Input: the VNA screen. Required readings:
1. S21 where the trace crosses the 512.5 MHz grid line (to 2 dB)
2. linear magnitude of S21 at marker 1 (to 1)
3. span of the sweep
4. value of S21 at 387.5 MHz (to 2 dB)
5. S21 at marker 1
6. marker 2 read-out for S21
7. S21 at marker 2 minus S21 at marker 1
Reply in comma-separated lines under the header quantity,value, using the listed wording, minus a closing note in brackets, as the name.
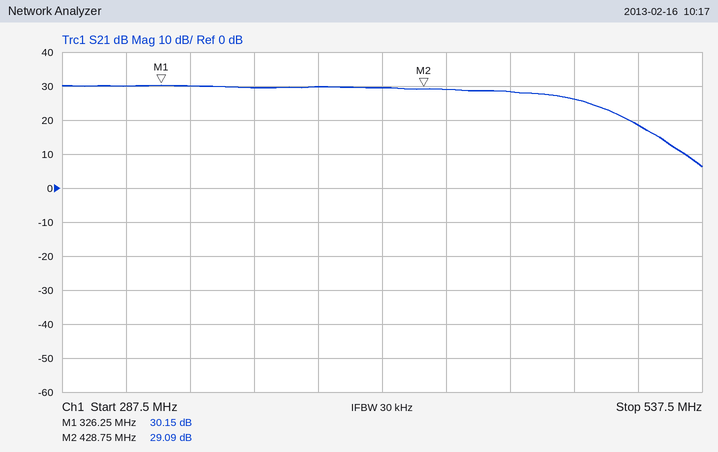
quantity,value
S21 where the trace crosses the 512.5 MHz grid line,18 dB
linear magnitude of S21 at marker 1,32
span of the sweep,250 MHz
value of S21 at 387.5 MHz,30 dB
S21 at marker 1,30.15 dB
marker 2 read-out for S21,29.09 dB
S21 at marker 2 minus S21 at marker 1,-1.06 dB
